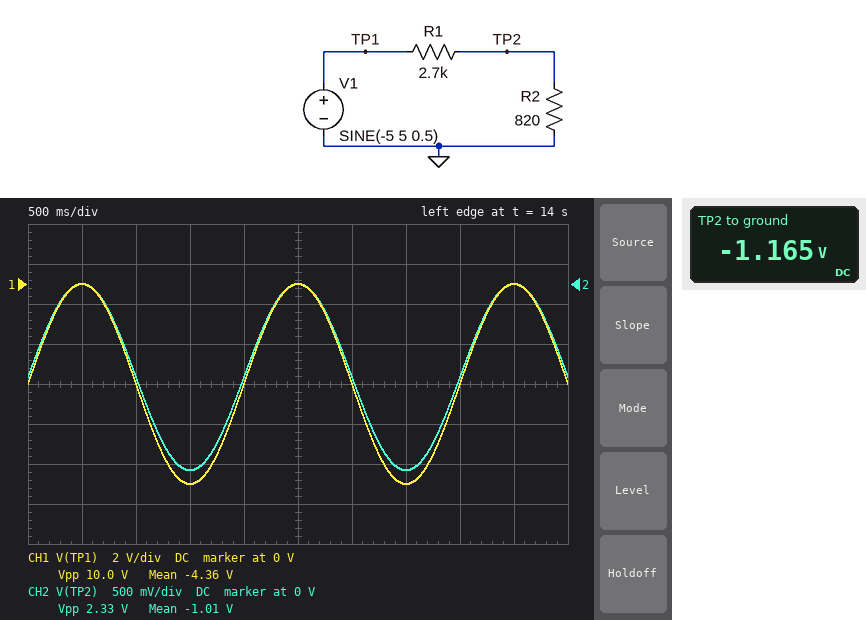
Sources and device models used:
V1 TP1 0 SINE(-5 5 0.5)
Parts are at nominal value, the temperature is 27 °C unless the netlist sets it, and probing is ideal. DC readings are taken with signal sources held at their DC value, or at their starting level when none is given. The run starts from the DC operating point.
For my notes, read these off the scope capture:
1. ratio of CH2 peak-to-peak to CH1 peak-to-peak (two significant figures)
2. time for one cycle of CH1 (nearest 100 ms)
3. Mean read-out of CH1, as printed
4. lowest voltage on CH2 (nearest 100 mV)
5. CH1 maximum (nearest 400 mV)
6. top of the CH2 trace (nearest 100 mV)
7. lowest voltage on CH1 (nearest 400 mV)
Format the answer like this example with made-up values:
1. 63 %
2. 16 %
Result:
1. 0.23
2. 2.0 s
3. -4.36 V
4. -2.3 V
5. 0 V
6. 0 V
7. -10.0 V
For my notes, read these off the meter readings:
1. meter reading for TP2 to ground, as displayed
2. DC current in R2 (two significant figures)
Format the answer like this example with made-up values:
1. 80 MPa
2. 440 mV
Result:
1. -1.165 V
2. 1.4 mA
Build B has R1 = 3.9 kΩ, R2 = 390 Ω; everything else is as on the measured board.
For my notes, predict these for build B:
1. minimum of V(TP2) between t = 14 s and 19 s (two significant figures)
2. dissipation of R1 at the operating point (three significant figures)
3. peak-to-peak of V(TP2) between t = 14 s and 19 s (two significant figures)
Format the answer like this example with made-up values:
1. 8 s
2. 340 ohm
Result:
1. -910 mV
2. 5.30 mW
3. 910 mV
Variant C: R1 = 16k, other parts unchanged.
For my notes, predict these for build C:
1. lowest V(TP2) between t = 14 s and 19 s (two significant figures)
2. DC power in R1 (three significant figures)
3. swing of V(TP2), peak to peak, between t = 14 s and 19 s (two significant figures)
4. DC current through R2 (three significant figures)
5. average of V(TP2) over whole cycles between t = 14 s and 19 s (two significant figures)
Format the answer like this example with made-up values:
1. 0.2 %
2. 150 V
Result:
1. -490 mV
2. 1.41 mW
3. 490 mV
4. 297 µA
5. -240 mV
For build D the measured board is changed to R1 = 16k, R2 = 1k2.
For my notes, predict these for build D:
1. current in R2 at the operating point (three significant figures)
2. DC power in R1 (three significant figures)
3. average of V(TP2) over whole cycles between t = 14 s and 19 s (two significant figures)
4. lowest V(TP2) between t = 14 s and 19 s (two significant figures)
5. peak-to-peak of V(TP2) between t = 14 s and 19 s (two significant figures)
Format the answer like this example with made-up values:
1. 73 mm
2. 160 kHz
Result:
1. 291 µA
2. 1.35 mW
3. -350 mV
4. -700 mV
5. 700 mV
